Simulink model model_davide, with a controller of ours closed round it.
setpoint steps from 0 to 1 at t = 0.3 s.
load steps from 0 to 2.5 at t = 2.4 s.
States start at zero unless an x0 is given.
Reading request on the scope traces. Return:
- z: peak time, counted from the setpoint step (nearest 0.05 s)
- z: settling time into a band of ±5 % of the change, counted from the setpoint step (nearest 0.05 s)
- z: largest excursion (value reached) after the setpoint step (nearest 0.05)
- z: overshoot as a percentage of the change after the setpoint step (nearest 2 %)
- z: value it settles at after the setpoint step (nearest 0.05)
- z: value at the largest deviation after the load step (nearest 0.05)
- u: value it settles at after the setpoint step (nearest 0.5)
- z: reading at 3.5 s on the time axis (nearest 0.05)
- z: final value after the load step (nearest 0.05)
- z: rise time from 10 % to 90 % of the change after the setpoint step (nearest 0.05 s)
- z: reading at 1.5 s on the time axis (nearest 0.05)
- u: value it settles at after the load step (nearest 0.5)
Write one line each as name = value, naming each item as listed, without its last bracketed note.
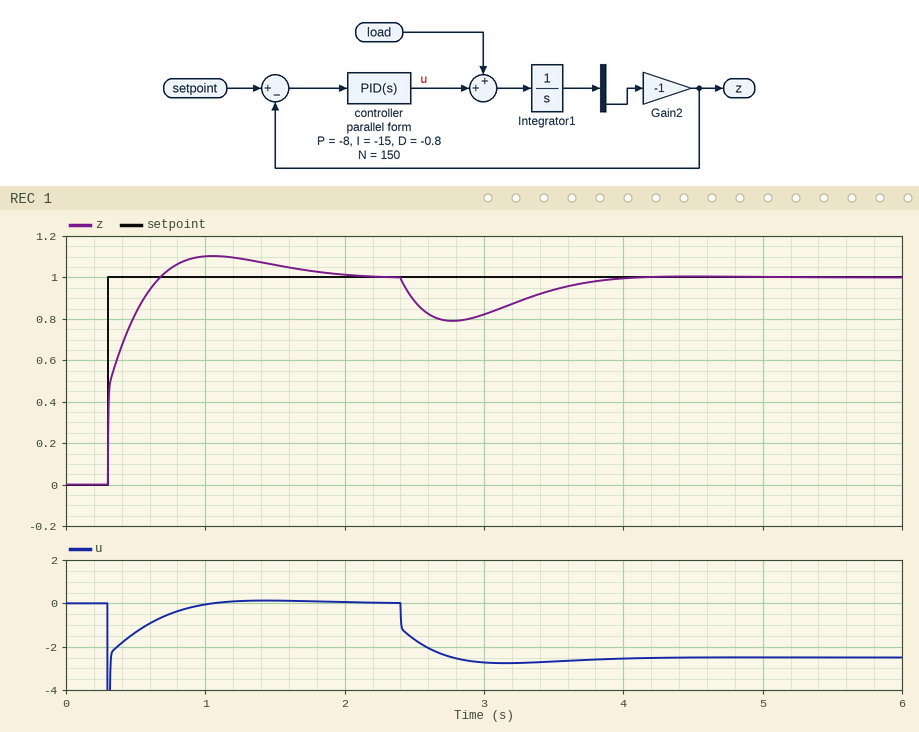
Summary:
z: peak time, counted from the setpoint step = 0.75 s
z: settling time into a band of ±5 % of the change, counted from the setpoint step = 1.30 s
z: largest excursion (value reached) after the setpoint step = 1.10
z: overshoot as a percentage of the change after the setpoint step = 10 %
z: value it settles at after the setpoint step = 1.00
z: value at the largest deviation after the load step = 0.80
u: value it settles at after the setpoint step = 0.0
z: reading at 3.5 s on the time axis = 0.95
z: final value after the load step = 1.00
z: rise time from 10 % to 90 % of the change after the setpoint step = 0.25 s
z: reading at 1.5 s on the time axis = 1.05
u: value it settles at after the load step = -2.5
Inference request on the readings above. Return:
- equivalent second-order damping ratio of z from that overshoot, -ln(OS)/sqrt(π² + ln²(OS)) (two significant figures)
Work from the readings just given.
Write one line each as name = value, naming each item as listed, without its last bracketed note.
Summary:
equivalent second-order damping ratio of z from that overshoot, -ln(OS)/sqrt(π² + ln²(OS)) = 0.59
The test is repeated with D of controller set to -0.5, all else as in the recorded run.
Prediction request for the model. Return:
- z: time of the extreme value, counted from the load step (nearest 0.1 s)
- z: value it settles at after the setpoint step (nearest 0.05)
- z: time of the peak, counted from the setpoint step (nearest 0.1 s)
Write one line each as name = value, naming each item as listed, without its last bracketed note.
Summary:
z: time of the extreme value, counted from the load step = 0.3 s
z: value it settles at after the setpoint step = 1.00
z: time of the peak, counted from the setpoint step = 0.7 s
